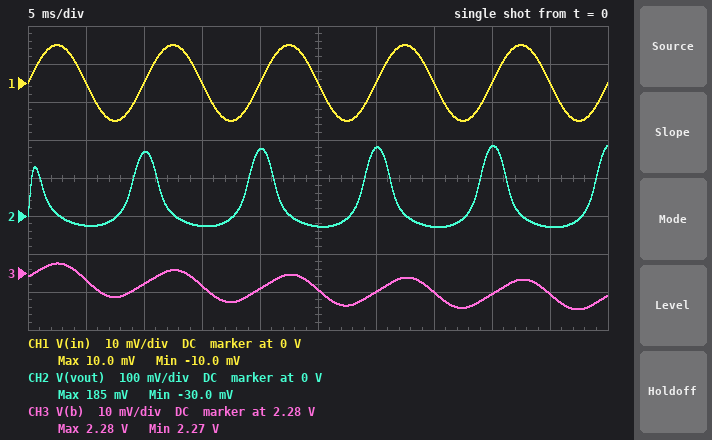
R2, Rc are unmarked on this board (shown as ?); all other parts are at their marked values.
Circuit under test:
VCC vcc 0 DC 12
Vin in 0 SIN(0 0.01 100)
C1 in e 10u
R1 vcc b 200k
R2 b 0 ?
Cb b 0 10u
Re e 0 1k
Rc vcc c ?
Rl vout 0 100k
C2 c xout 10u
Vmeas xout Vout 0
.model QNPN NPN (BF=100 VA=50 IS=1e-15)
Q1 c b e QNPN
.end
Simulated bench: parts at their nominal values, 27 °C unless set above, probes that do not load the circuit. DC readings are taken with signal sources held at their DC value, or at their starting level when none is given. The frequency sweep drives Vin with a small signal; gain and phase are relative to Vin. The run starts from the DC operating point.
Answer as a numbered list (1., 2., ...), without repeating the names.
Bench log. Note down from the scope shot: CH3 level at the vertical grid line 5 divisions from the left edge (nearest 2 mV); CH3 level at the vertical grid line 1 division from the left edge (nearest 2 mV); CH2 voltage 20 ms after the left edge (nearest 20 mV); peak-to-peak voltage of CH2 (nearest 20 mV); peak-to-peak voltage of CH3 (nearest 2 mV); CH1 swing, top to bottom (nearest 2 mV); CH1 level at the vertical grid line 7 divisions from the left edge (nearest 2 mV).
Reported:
1. 2.276 V
2. 2.278 V
3. 180 mV
4. 220 mV
5. 12 mV
6. 20 mV
7. 0 V
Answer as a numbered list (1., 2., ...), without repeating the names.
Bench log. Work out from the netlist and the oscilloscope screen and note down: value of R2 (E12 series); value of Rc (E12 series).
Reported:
1. 150 kΩ
2. 6.8 kΩ
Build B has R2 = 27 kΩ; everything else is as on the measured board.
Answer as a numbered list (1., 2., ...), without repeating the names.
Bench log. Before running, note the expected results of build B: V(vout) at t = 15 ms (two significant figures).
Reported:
1. -350 mV
